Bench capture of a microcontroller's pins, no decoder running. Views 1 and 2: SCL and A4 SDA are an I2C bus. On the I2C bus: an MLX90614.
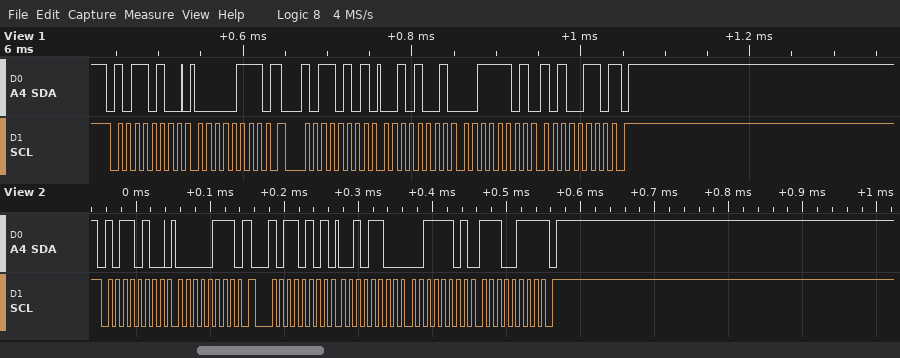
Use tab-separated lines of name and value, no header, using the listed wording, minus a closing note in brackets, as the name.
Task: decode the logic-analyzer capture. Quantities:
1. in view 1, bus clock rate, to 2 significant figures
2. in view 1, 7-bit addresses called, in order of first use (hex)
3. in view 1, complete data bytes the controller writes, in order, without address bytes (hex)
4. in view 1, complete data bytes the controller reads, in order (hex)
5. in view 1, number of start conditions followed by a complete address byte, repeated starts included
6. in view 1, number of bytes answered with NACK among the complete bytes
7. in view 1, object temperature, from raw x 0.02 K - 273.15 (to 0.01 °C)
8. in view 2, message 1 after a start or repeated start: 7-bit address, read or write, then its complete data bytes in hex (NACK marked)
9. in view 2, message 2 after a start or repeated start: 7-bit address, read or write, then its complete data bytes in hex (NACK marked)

in view 1, bus clock rate, to 2 significant figures	100 kHz
in view 1, 7-bit addresses called, in order of first use	0x5A
in view 1, complete data bytes the controller writes, in order, without address bytes	07
in view 1, complete data bytes the controller reads, in order	29 3D A6
in view 1, number of start conditions followed by a complete address byte, repeated starts included	2
in view 1, number of bytes answered with NACK among the complete bytes	1
in view 1, object temperature, from raw x 0.02 K - 273.15	39.99 °C
in view 2, message 1 after a start or repeated start: 7-bit address, read or write, then its complete data bytes in hex	0x5A write: 07
in view 2, message 2 after a start or repeated start: 7-bit address, read or write, then its complete data bytes in hex	0x5A read: 2C 3D E7 NACK
